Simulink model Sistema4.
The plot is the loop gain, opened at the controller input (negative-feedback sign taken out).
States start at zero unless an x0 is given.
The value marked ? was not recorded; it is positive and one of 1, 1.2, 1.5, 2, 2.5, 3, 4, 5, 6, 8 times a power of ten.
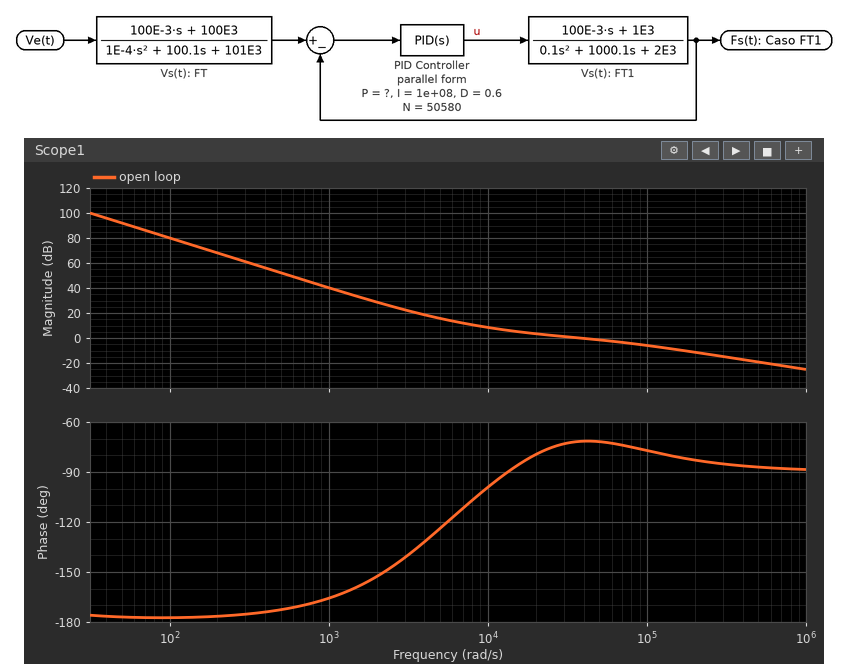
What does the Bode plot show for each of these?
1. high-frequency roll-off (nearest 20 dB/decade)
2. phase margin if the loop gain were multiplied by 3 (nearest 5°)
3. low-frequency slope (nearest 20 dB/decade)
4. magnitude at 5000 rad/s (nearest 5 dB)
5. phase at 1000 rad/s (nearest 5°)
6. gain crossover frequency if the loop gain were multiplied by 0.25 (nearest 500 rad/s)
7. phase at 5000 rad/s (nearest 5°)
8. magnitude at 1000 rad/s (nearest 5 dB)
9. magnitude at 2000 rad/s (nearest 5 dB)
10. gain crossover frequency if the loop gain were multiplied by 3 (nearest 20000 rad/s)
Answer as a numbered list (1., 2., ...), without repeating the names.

1. -20 dB/decade
2. 100°
3. -40 dB/decade
4. 15 dB
5. -165°
6. 7000 rad/s
7. -125°
8. 40 dB
9. 30 dB
10. 160000 rad/s
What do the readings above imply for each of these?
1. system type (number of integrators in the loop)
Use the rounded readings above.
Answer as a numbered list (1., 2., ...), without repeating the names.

1. 2
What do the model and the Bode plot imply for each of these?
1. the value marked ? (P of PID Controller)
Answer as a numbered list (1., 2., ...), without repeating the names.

1. 25000
